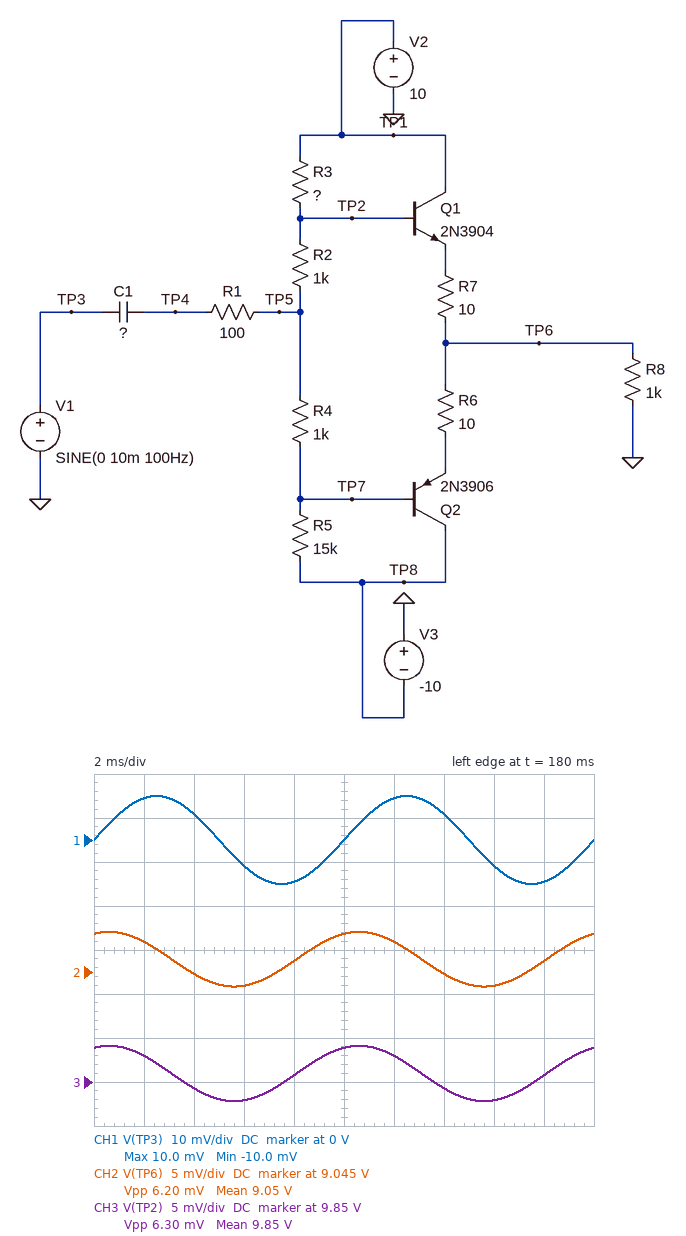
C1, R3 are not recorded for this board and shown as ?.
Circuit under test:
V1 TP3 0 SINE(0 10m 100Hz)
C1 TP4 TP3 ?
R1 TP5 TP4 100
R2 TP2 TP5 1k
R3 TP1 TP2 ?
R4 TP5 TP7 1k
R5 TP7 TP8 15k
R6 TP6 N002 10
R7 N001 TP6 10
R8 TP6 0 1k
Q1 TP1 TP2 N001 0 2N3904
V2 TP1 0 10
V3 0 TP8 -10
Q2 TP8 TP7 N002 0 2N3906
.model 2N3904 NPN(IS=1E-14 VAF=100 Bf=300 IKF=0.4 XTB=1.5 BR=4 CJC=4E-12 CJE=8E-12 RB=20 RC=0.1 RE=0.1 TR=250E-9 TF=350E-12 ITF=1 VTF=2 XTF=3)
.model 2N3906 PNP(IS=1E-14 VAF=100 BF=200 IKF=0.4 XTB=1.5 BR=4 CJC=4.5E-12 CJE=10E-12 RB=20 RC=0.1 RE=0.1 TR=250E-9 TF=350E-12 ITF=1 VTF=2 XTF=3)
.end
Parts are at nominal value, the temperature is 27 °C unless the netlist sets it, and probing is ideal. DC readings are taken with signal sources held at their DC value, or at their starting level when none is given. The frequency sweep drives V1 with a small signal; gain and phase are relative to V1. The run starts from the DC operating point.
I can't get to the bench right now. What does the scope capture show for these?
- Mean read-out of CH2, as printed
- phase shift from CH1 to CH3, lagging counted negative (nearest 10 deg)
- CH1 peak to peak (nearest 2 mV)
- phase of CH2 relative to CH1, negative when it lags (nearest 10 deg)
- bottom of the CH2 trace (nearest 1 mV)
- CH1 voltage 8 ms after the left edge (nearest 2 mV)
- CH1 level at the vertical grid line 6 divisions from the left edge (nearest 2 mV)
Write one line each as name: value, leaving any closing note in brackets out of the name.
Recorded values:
Mean read-out of CH2, as printed: 9.05 V
phase shift from CH1 to CH3, lagging counted negative: 70 deg
CH1 peak to peak: 20 mV
phase of CH2 relative to CH1, negative when it lags: 70 deg
bottom of the CH2 trace: 9.043 V
CH1 voltage 8 ms after the left edge: -10 mV
CH1 level at the vertical grid line 6 divisions from the left edge: 10 mV
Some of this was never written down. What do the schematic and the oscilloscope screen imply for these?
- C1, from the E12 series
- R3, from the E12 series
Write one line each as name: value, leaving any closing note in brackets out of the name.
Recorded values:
C1, from the E12 series: 120 nF
R3, from the E12 series: 6.8 kΩ
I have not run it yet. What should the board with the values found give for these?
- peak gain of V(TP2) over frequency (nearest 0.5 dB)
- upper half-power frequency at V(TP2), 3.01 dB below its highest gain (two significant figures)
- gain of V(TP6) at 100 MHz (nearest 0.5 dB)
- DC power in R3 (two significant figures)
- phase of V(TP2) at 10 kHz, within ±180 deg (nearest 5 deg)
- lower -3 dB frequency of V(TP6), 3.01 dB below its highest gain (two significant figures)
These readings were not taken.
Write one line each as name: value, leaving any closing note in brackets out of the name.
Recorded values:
peak gain of V(TP2) over frequency: -1.5 dB
upper half-power frequency at V(TP2), 3.01 dB below its highest gain: 36 MHz
gain of V(TP6) at 100 MHz: -10.5 dB
DC power in R3: 3.3 µW
phase of V(TP2) at 10 kHz, within ±180 deg: 0 deg
lower -3 dB frequency of V(TP6), 3.01 dB below its highest gain: 250 Hz
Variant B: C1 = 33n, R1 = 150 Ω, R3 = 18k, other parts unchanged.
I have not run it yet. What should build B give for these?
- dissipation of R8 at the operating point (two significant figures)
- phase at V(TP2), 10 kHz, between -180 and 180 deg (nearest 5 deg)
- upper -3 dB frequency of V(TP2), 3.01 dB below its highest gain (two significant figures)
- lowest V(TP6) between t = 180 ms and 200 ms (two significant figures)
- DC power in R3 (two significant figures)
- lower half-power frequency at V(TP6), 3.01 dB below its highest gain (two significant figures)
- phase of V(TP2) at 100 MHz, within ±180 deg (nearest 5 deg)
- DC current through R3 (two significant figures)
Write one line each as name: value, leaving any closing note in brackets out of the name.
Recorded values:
dissipation of R8 at the operating point: 80 mW
phase at V(TP2), 10 kHz, between -180 and 180 deg: 5 deg
upper -3 dB frequency of V(TP2), 3.01 dB below its highest gain: 32 MHz
lowest V(TP6) between t = 180 ms and 200 ms: 8.9 V
DC power in R3: 3.9 µW
lower half-power frequency at V(TP6), 3.01 dB below its highest gain: 560 Hz
phase of V(TP2) at 100 MHz, within ±180 deg: -70 deg
DC current through R3: 15 µA
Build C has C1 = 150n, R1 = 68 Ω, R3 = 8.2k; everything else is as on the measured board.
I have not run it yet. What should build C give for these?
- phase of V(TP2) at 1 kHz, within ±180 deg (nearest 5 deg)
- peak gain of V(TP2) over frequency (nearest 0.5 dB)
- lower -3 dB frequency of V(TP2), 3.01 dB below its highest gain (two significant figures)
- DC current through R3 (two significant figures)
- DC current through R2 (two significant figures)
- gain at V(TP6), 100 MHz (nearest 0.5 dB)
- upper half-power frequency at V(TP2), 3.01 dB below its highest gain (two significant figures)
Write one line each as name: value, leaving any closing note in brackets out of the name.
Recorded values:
phase of V(TP2) at 1 kHz, within ±180 deg: 10 deg
peak gain of V(TP2) over frequency: -1.0 dB
lower -3 dB frequency of V(TP2), 3.01 dB below its highest gain: 180 Hz
DC current through R3: 21 µA
DC current through R2: 10 µA
gain at V(TP6), 100 MHz: -10.0 dB
upper half-power frequency at V(TP2), 3.01 dB below its highest gain: 38 MHz
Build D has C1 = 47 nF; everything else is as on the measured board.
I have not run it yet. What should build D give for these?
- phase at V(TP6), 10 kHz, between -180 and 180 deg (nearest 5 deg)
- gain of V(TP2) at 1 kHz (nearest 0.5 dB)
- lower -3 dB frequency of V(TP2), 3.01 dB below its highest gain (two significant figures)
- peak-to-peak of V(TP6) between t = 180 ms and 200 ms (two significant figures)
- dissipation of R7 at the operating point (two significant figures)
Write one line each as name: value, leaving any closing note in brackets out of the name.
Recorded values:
phase at V(TP6), 10 kHz, between -180 and 180 deg: 5 deg
gain of V(TP2) at 1 kHz: -3.0 dB
lower -3 dB frequency of V(TP2), 3.01 dB below its highest gain: 640 Hz
peak-to-peak of V(TP6) between t = 180 ms and 200 ms: 2.6 mV
dissipation of R7 at the operating point: 820 µW
